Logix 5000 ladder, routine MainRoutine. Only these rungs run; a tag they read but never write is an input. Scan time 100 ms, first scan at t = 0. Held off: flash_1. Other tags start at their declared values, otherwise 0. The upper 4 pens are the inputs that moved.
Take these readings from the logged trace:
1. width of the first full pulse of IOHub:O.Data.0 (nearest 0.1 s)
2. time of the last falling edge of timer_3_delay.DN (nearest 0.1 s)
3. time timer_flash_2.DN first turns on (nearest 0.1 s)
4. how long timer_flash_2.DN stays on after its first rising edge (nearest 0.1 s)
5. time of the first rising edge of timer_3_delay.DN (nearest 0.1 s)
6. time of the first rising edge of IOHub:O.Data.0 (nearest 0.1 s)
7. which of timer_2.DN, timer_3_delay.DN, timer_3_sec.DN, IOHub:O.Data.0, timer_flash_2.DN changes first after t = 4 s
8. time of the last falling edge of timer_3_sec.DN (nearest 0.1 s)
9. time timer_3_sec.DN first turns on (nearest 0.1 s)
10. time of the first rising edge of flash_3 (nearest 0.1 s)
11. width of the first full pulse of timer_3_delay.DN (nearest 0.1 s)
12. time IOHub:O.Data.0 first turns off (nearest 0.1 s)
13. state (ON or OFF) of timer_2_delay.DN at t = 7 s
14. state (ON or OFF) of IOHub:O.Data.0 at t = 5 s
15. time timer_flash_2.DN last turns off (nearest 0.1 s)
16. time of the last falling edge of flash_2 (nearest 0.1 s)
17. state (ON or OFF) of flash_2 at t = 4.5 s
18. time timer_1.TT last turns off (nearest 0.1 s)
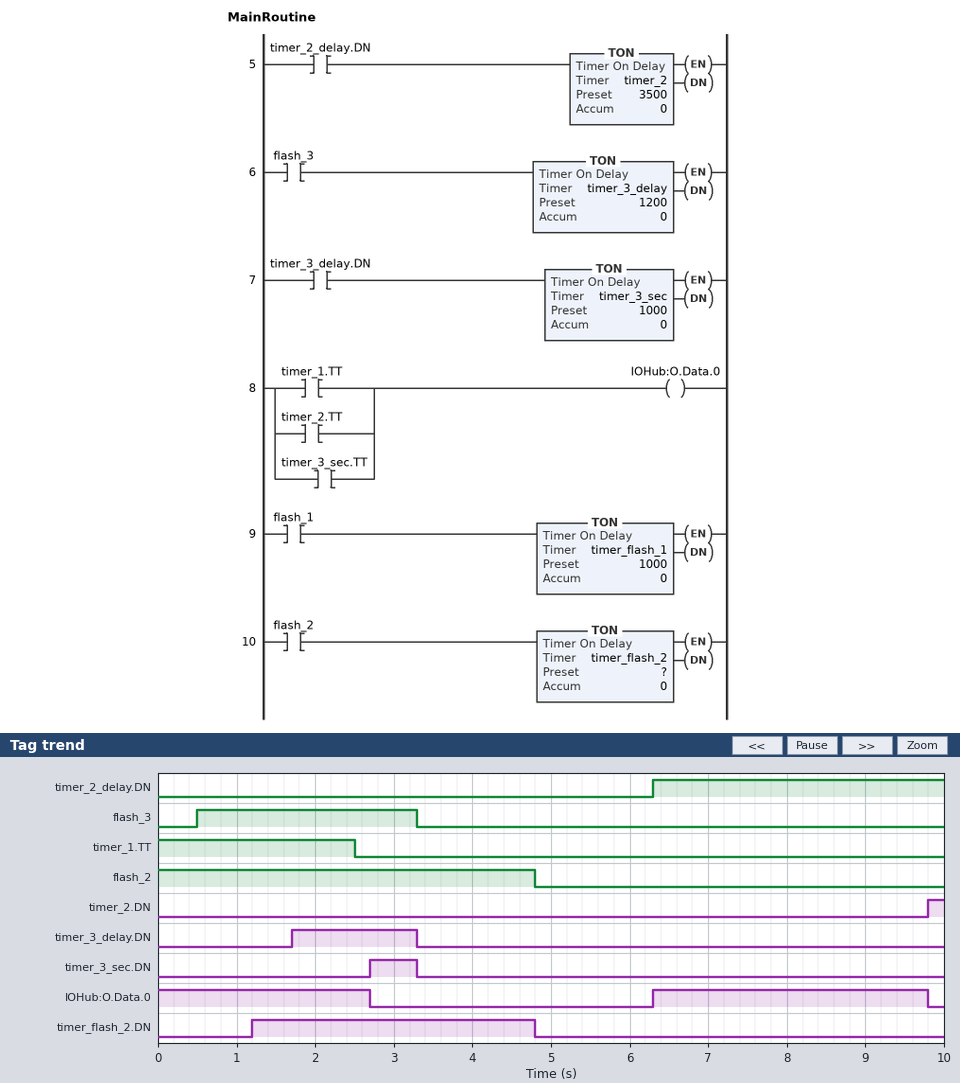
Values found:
3.5 s
3.3 s
1.2 s
3.6 s
1.7 s
6.3 s
timer_flash_2.DN
3.3 s
2.7 s
0.5 s
1.6 s
2.7 s
ON
OFF
4.8 s
4.8 s
ON
2.5 s
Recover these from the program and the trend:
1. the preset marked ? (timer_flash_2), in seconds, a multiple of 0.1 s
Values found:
1.2 s
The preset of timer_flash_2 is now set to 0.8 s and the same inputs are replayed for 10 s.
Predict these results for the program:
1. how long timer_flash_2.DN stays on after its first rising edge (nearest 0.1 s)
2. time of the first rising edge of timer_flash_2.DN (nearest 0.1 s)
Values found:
4.0 s
0.8 s
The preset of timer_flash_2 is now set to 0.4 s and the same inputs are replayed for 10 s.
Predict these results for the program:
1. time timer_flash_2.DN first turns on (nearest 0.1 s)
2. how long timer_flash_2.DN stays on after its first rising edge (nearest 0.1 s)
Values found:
0.4 s
4.4 s
